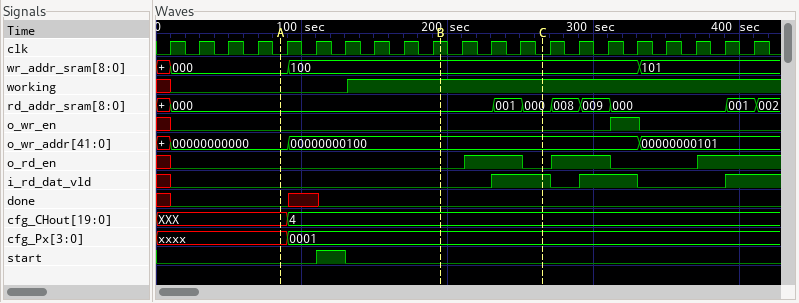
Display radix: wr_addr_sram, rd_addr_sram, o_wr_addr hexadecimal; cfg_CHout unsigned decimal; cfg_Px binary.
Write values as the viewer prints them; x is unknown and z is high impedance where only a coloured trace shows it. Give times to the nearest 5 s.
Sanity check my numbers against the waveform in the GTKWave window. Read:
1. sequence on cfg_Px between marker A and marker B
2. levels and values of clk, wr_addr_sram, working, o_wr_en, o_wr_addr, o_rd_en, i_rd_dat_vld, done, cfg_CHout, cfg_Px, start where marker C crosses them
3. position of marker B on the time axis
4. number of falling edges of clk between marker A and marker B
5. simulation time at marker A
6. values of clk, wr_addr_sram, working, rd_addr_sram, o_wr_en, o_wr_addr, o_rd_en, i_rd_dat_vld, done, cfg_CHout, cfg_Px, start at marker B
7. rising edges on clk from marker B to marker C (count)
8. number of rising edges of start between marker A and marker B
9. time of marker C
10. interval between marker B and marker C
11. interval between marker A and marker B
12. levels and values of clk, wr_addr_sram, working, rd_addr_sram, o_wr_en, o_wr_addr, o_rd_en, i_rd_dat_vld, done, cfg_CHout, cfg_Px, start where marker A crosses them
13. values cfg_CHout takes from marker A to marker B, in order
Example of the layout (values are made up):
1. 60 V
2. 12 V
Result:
1. xxxx, 0001
2. clk=0, wr_addr_sram=100, working=1, o_wr_en=0, o_wr_addr=00000000100, o_rd_en=0, i_rd_dat_vld=1, done=0, cfg_CHout=4, cfg_Px=0001, start=0
3. 195 s
4. 5
5. 85 s
6. clk=1, wr_addr_sram=100, working=1, rd_addr_sram=000, o_wr_en=0, o_wr_addr=00000000100, o_rd_en=0, i_rd_dat_vld=0, done=0, cfg_CHout=4, cfg_Px=0001, start=0
7. 3
8. 1
9. 265 s
10. 70 s
11. 110 s
12. clk=0, wr_addr_sram=000, working=0, rd_addr_sram=000, o_wr_en=0, o_wr_addr=00000000000, o_rd_en=0, i_rd_dat_vld=0, done=0, cfg_CHout=XXX, cfg_Px=xxxx, start=0
13. XXX, 4
